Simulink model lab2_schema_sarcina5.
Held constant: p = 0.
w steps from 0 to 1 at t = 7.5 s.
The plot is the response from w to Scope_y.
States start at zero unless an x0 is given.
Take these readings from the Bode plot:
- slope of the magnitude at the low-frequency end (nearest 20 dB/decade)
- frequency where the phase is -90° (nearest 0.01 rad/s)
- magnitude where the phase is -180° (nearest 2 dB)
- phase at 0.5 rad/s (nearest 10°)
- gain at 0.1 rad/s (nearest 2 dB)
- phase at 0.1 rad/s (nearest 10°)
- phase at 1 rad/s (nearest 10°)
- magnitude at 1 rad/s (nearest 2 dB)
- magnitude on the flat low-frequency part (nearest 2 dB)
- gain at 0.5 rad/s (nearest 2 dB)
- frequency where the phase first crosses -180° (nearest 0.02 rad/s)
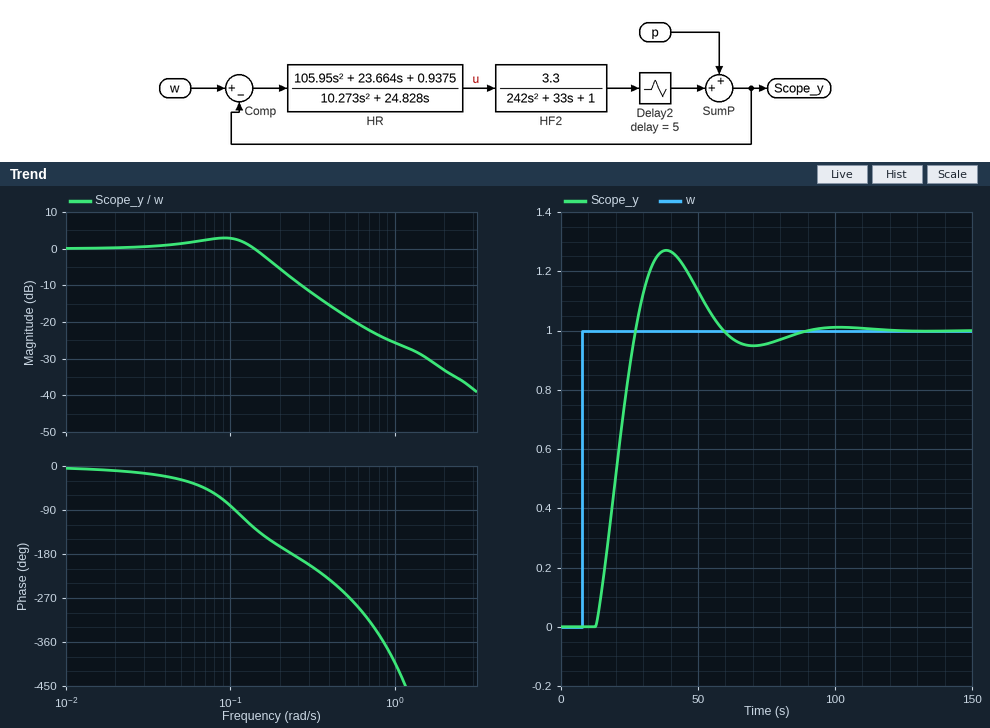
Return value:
0 dB/decade
0.11 rad/s
-8 dB
-260°
2 dB
-80°
-400°
-26 dB
0 dB
-18 dB
0.24 rad/s
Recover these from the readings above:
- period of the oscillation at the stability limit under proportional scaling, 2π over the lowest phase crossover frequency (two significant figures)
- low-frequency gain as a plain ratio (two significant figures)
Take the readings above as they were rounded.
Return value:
26 s
1.0
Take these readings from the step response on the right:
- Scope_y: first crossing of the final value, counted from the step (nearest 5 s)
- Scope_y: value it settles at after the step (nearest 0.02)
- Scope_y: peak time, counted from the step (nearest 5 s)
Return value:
20 s
1.00
30 s
